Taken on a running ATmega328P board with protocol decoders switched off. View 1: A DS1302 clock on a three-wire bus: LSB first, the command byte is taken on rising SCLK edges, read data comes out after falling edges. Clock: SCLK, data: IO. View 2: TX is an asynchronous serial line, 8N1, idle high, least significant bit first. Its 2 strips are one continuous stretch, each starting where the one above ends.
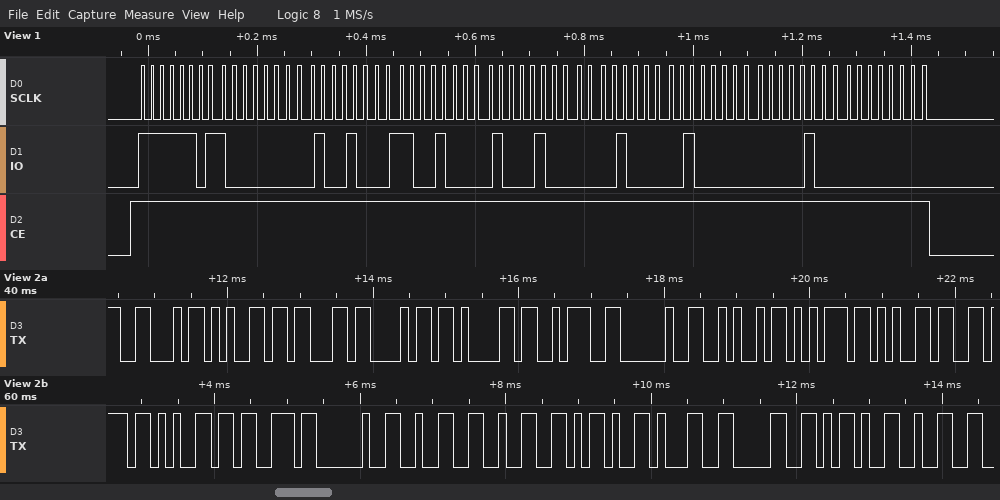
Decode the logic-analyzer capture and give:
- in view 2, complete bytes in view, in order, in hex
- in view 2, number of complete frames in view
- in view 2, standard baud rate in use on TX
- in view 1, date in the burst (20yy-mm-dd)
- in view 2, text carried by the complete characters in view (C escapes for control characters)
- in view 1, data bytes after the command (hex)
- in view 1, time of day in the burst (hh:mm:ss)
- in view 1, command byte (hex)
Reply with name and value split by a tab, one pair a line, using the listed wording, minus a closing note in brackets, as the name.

in view 2, complete bytes in view, in order, in hex	46 65 63 68 61 3A 20 4A 75 65 76 65 73 20 32 32 2D 31 30 2D 32
in view 2, number of complete frames in view	21
in view 2, standard baud rate in use on TX	9600 baud
in view 1, date in the burst	2020-10-22
in view 2, text carried by the complete characters in view	"Fecha: Jueves 22-10-2"
in view 1, data bytes after the command	01 12 13 22 10 04 20 00
in view 1, time of day in the burst	13:12:01
in view 1, command byte	0xBF
